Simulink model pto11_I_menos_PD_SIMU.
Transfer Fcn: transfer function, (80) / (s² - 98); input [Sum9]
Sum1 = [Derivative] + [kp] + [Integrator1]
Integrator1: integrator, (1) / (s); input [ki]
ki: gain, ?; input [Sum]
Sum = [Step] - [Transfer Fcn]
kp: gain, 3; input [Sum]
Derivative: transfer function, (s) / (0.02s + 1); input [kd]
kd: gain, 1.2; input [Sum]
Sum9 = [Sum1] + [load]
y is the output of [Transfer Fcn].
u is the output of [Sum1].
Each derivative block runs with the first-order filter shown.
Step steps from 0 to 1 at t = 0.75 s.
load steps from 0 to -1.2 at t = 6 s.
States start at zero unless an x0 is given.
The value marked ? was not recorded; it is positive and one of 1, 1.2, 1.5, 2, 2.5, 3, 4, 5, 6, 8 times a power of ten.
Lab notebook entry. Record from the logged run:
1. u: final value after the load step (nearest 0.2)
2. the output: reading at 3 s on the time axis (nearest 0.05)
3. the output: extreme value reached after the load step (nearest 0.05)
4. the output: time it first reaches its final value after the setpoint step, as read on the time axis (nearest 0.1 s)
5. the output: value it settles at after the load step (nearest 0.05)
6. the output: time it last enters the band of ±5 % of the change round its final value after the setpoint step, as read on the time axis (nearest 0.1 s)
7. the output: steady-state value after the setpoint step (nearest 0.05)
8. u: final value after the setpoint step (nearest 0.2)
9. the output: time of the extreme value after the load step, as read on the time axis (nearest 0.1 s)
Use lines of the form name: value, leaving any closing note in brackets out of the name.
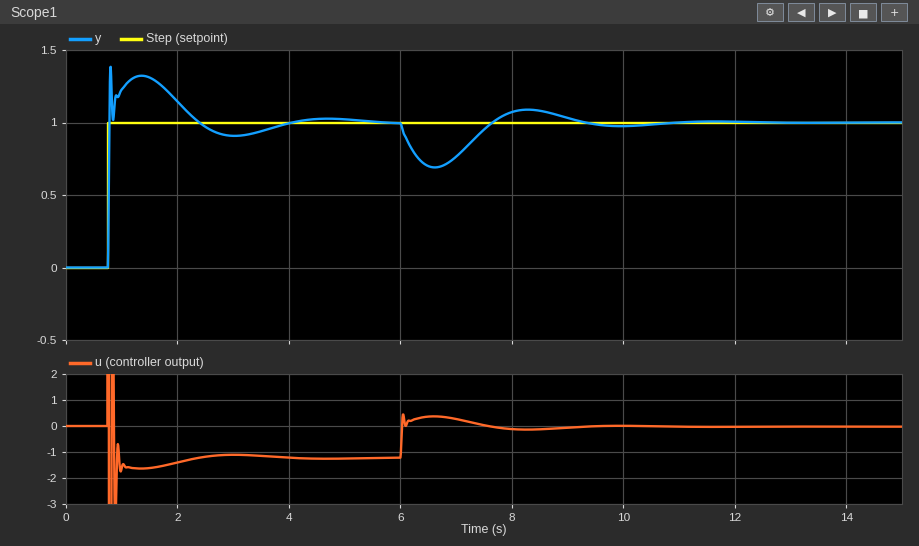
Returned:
u: final value after the load step: 0.0
the output: reading at 3 s on the time axis: 0.90
the output: extreme value reached after the load step: 0.70
the output: time it first reaches its final value after the setpoint step, as read on the time axis: 0.8 s
the output: value it settles at after the load step: 1.00
the output: time it last enters the band of ±5 % of the change round its final value after the setpoint step, as read on the time axis: 3.6 s
the output: steady-state value after the setpoint step: 1.00
u: final value after the setpoint step: -1.2
the output: time of the extreme value after the load step, as read on the time axis: 6.6 s
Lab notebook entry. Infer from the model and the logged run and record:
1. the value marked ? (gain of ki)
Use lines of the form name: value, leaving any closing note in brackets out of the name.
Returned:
the value marked ?: 5
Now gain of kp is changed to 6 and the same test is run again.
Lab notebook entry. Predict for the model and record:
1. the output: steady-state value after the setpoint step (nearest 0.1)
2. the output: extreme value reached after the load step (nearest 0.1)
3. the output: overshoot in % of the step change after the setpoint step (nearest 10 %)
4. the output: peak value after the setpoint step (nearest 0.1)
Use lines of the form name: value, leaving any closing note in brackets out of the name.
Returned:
the output: steady-state value after the setpoint step: 1.0
the output: extreme value reached after the load step: 0.8
the output: overshoot in % of the step change after the setpoint step: 40 %
the output: peak value after the setpoint step: 1.4
